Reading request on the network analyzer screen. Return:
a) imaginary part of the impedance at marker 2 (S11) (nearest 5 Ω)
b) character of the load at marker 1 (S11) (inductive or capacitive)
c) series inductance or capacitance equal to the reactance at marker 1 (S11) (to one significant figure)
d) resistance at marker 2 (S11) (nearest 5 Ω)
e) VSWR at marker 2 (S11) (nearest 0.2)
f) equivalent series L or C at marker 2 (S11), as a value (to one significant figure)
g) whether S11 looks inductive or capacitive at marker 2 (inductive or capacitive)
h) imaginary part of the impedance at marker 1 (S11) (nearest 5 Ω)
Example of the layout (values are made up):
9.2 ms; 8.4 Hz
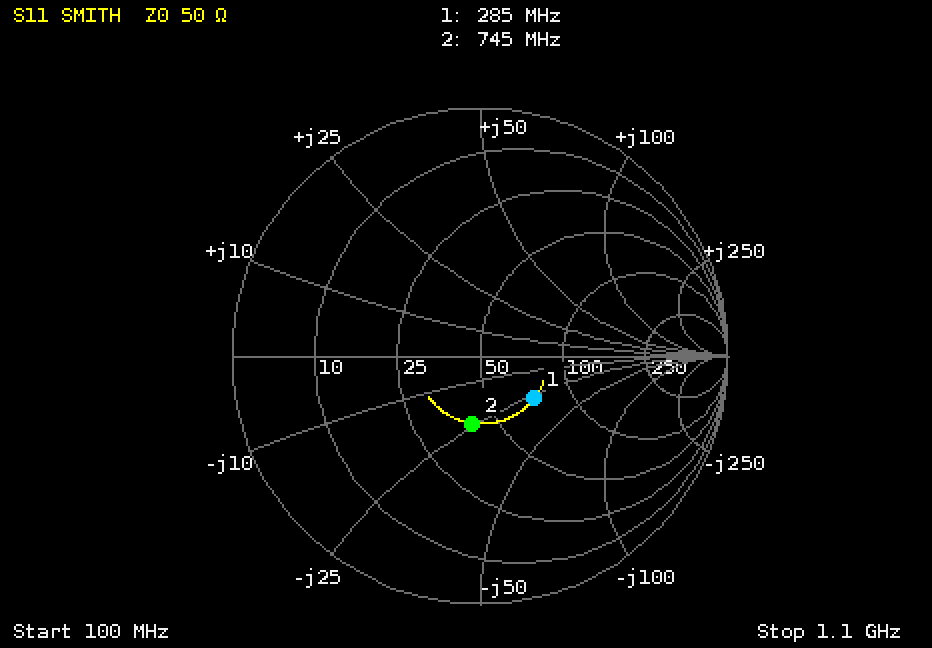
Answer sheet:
-25 Ω; capacitive; 20 pF; 40 Ω; 1.8; 9 pF; capacitive; -25 Ω
